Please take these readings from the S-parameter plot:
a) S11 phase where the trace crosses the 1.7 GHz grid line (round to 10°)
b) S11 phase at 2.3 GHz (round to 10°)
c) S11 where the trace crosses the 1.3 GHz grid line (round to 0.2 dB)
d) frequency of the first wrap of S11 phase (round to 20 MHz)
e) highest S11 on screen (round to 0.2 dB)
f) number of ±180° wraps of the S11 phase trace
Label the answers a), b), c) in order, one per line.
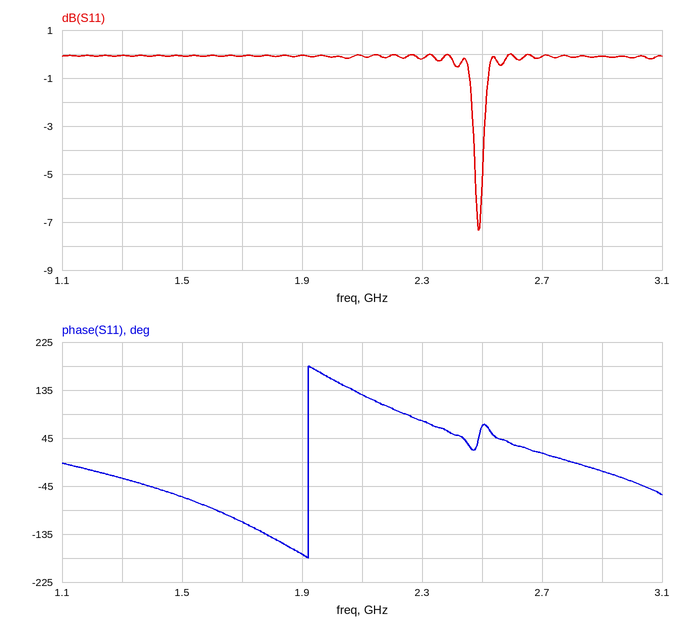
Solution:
a) -110°
b) 80°
c) 0.0 dB
d) 1.92 GHz
e) 0.0 dB
f) 1
